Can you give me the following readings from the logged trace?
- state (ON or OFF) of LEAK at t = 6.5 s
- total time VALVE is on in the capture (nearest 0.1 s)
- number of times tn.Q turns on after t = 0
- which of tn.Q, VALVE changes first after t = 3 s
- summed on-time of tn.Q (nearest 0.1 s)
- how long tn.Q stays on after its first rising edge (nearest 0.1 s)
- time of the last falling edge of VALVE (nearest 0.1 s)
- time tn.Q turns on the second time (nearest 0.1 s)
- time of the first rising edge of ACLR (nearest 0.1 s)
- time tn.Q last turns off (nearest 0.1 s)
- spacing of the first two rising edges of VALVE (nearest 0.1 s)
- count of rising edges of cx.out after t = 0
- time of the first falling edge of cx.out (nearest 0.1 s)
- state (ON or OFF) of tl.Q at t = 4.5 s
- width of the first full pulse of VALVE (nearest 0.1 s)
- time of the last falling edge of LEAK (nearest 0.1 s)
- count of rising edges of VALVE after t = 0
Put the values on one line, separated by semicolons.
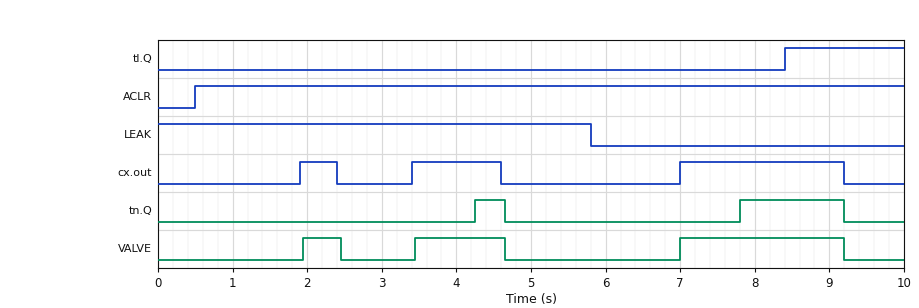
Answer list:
OFF; 3.9 s; 2; VALVE; 1.8 s; 0.4 s; 9.2 s; 7.8 s; 0.5 s; 9.2 s; 1.5 s; 3; 2.4 s; OFF; 0.5 s; 5.8 s; 3
